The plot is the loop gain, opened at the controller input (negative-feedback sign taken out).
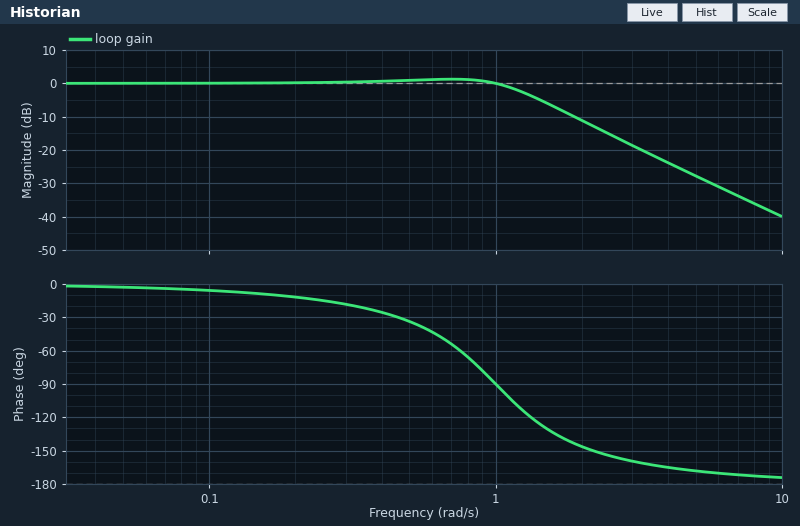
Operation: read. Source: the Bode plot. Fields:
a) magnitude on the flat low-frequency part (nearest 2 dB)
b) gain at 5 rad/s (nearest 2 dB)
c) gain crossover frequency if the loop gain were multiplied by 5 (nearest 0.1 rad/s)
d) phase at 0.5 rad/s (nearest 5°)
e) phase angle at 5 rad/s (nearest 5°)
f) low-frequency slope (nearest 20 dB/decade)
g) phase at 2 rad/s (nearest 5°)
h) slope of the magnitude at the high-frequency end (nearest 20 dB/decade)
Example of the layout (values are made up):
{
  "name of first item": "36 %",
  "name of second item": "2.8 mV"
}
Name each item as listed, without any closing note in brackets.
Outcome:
{
  "magnitude on the flat low-frequency part": "0 dB",
  "gain at 5 rad/s": "-28 dB",
  "gain crossover frequency if the loop gain were multiplied by 5": "2.3 rad/s",
  "phase at 0.5 rad/s": "-35°",
  "phase angle at 5 rad/s": "-170°",
  "low-frequency slope": "0 dB/decade",
  "phase at 2 rad/s": "-145°",
  "slope of the magnitude at the high-frequency end": "-40 dB/decade"
}
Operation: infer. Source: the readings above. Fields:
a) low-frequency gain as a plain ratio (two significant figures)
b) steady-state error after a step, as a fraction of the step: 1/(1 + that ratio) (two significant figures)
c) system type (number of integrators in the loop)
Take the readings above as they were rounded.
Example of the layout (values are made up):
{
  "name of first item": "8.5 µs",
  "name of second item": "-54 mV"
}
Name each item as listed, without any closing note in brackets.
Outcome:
{
  "low-frequency gain as a plain ratio": "1.0",
  "steady-state error after a step, as a fraction of the step: 1/(1 + that ratio)": "0.50",
  "system type": "0"
}
